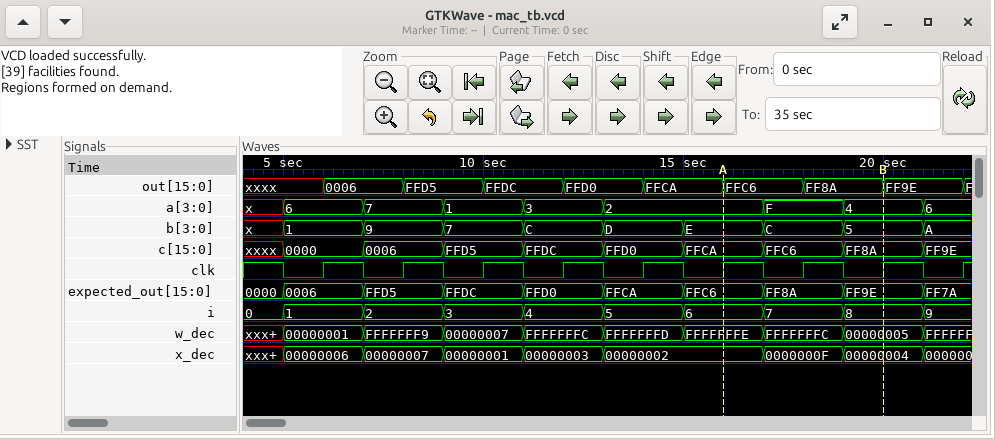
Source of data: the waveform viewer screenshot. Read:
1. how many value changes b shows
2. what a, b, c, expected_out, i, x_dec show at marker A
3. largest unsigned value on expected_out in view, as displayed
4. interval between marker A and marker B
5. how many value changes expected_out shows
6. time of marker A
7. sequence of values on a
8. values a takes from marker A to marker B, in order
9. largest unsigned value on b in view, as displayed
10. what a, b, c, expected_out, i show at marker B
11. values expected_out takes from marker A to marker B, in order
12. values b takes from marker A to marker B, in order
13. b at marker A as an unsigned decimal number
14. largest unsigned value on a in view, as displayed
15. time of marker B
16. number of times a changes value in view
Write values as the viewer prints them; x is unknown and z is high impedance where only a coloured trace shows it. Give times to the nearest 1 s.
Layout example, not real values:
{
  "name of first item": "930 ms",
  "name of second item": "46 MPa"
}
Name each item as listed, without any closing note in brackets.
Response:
{
  "how many value changes b shows": "9",
  "what a, b, c, expected_out, i, x_dec show at marker A": "a=2, b=E, c=FFCA, expected_out=FFC6, i=6, x_dec=00000002",
  "largest unsigned value on expected_out in view, as displayed": "FFDC",
  "interval between marker A and marker B": "4 s",
  "how many value changes expected_out shows": "9",
  "time of marker A": "16 s",
  "sequence of values on a": "x, 6, 7, 1, 3, 2, F, 4, 6",
  "values a takes from marker A to marker B, in order": "2, F, 4",
  "largest unsigned value on b in view, as displayed": "E",
  "what a, b, c, expected_out, i show at marker B": "a=4, b=5, c=FF8A, expected_out=FF9E, i=8",
  "values expected_out takes from marker A to marker B, in order": "FFC6, FF8A, FF9E",
  "values b takes from marker A to marker B, in order": "E, C, 5",
  "b at marker A as an unsigned decimal number": "14",
  "largest unsigned value on a in view, as displayed": "F",
  "time of marker B": "20 s",
  "number of times a changes value in view": "8"
}
